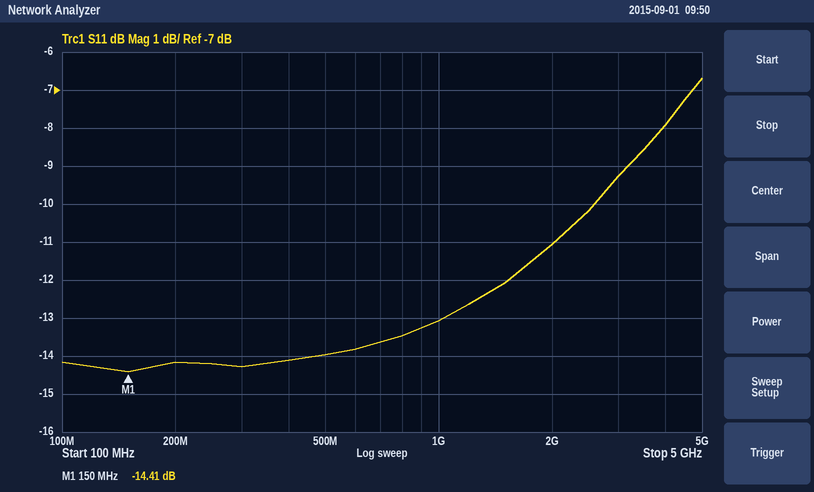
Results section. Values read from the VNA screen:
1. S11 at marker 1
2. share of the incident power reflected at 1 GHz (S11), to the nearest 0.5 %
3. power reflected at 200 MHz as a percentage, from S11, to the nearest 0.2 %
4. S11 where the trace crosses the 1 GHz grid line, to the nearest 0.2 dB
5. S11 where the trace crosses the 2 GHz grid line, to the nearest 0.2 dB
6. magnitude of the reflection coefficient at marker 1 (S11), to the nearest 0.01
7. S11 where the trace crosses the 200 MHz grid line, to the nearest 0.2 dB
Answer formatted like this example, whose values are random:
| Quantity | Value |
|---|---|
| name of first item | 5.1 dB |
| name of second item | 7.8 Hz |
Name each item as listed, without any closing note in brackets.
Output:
| Quantity | Value |
|---|---|
| S11 at marker 1 | -14.41 dB |
| share of the incident power reflected at 1 GHz (S11), to the nearest 0.5 % | 5.0 % |
| power reflected at 200 MHz as a percentage, from S11, to the nearest 0.2 % | 3.8 % |
| S11 where the trace crosses the 1 GHz grid line, to the nearest 0.2 dB | -13.0 dB |
| S11 where the trace crosses the 2 GHz grid line, to the nearest 0.2 dB | -11.0 dB |
| magnitude of the reflection coefficient at marker 1 (S11), to the nearest 0.01 | 0.19 |
| S11 where the trace crosses the 200 MHz grid line, to the nearest 0.2 dB | -14.2 dB |
